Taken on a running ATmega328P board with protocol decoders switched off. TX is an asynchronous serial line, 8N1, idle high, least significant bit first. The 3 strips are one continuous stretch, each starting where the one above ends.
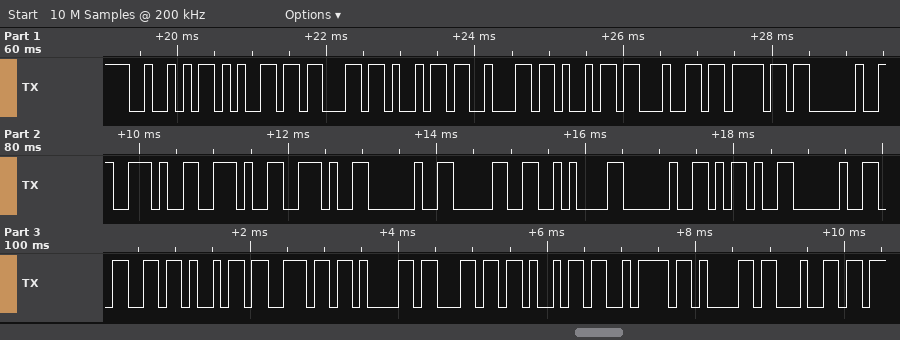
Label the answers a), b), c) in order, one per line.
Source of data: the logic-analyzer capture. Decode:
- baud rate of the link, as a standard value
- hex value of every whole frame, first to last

a) 9600 baud
b) 0x52 0x65 0x63 0x69 0x62 0x69 0x64 0x6F 0x20 0x2E 0x2E 0x2E 0x20 0x30 0x0A 0x20 0x2D 0x20 0x66 0x69 0x6E 0x61 0x6C 0x69 0x7A 0x61 0x64
